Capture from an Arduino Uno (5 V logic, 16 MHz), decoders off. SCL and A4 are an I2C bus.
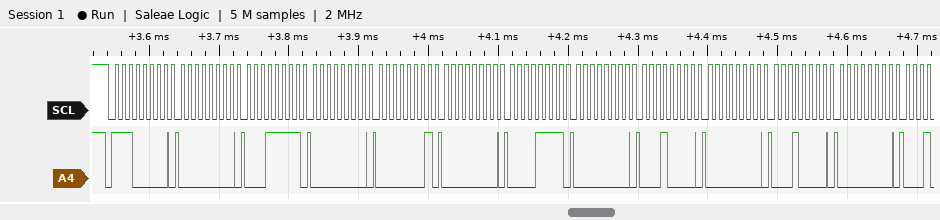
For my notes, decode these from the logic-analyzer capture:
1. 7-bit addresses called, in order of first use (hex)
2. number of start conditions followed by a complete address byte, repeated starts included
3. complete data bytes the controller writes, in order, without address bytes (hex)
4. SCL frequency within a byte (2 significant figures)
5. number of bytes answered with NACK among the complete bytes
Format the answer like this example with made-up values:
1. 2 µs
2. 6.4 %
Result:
1. 0x70
2. 1
3. 00 1F 00 01 00 0F 00 10 00 10 00
4. 100 kHz
5. 0
